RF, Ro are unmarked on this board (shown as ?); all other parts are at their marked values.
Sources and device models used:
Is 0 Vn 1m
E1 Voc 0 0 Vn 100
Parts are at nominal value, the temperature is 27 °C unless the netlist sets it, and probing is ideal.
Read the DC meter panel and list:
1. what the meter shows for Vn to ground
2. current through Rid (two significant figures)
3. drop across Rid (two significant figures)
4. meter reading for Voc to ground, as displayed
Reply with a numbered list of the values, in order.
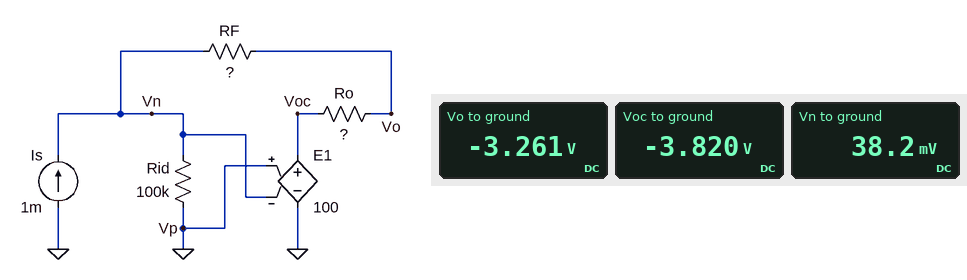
1. 38.2 mV
2. 380 nA
3. 38 mV
4. -3.820 V
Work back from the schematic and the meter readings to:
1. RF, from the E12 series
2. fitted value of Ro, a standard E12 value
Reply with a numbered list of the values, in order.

1. 3.3 kΩ
2. 560 Ω
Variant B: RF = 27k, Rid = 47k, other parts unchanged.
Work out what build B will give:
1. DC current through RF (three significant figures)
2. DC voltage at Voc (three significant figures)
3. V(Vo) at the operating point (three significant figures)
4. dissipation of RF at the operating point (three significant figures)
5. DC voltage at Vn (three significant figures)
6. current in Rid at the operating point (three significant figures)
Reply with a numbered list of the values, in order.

1. 994 µA
2. -27.1 V
3. -26.6 V
4. 26.7 mW
5. 271 mV
6. 5.77 µA
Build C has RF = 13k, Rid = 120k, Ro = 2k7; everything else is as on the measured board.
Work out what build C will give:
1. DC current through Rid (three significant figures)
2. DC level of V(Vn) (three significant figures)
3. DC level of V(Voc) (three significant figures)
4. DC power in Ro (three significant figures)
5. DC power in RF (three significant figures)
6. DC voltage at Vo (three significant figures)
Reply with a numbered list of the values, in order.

1. 1.29 µA
2. 155 mV
3. -15.5 V
4. 2.69 mW
5. 13.0 mW
6. -12.8 V
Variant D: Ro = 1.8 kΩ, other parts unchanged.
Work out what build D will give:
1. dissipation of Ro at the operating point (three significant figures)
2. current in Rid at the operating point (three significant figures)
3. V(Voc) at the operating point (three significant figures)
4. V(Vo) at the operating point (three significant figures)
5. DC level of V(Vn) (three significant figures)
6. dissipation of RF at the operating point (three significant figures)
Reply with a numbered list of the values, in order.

1. 1.80 mW
2. 505 nA
3. -5.05 V
4. -3.25 V
5. 50.5 mV
6. 3.30 mW
